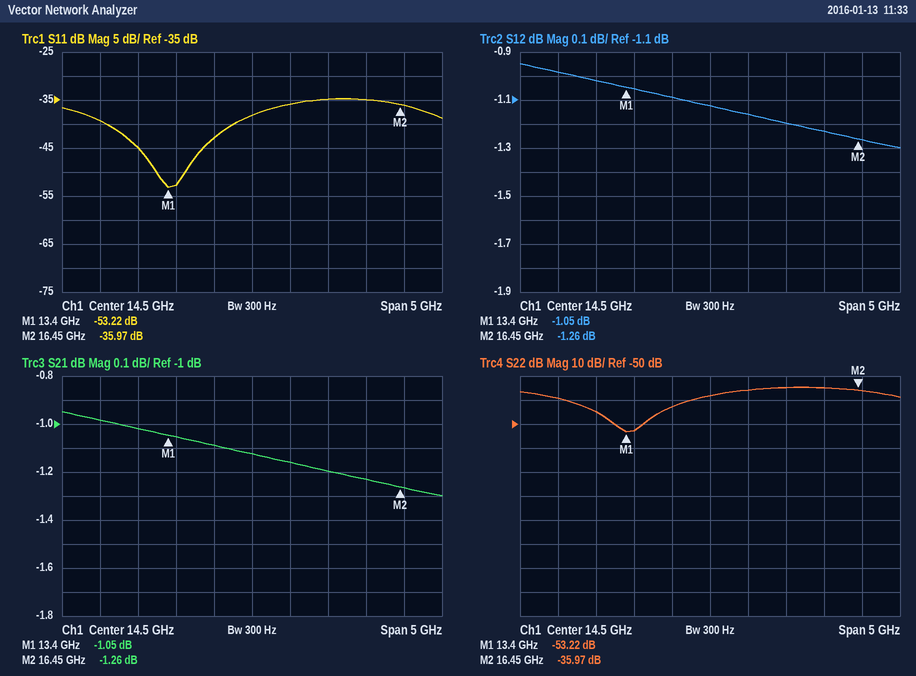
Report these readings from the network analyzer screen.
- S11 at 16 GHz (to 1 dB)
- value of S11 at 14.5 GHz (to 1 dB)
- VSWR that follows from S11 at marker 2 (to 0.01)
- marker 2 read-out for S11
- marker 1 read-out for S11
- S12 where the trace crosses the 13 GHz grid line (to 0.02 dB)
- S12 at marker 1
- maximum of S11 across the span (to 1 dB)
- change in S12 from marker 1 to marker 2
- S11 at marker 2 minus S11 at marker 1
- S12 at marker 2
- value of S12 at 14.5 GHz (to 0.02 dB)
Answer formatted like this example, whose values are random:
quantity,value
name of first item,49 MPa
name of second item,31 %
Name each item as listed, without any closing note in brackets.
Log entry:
quantity,value
S11 at 16 GHz,-35 dB
value of S11 at 14.5 GHz,-38 dB
VSWR that follows from S11 at marker 2,1.03
marker 2 read-out for S11,-35.97 dB
marker 1 read-out for S11,-53.22 dB
S12 where the trace crosses the 13 GHz grid line,-1.02 dB
S12 at marker 1,-1.05 dB
maximum of S11 across the span,-35 dB
change in S12 from marker 1 to marker 2,-0.21 dB
S11 at marker 2 minus S11 at marker 1,17.25 dB
S12 at marker 2,-1.26 dB
value of S12 at 14.5 GHz,-1.12 dB
